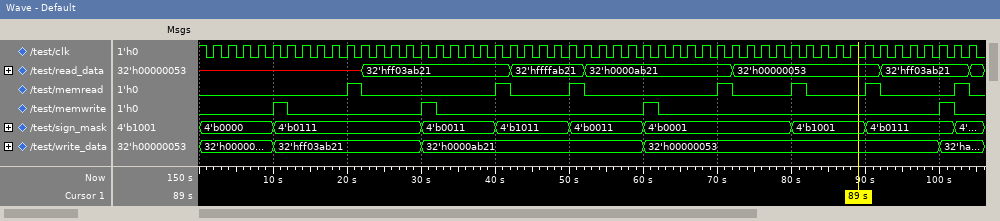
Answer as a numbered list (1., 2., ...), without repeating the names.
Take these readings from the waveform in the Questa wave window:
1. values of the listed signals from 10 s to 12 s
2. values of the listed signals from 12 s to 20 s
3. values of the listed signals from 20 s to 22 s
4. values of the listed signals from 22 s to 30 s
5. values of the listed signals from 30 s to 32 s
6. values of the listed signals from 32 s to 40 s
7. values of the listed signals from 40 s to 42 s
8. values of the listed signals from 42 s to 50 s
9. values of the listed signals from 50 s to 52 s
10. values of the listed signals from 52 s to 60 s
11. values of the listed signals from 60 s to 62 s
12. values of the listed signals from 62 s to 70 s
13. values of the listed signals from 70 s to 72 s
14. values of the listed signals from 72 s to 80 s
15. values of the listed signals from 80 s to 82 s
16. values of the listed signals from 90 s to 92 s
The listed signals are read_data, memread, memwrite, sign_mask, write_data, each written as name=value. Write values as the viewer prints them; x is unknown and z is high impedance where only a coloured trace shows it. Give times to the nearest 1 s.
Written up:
1. read_data=x, memread=0, memwrite=1, sign_mask=4'b0111, write_data=32'hff03ab21
2. read_data=x, memread=0, memwrite=0, sign_mask=4'b0111, write_data=32'hff03ab21
3. read_data=x, memread=1, memwrite=0, sign_mask=4'b0111, write_data=32'hff03ab21
4. read_data=32'hff03ab21, memread=0, memwrite=0, sign_mask=4'b0111, write_data=32'hff03ab21
5. read_data=32'hff03ab21, memread=0, memwrite=1, sign_mask=4'b0011, write_data=32'h0000ab21
6. read_data=32'hff03ab21, memread=0, memwrite=0, sign_mask=4'b0011, write_data=32'h0000ab21
7. read_data=32'hff03ab21, memread=1, memwrite=0, sign_mask=4'b1011, write_data=32'h0000ab21
8. read_data=32'hffffab21, memread=0, memwrite=0, sign_mask=4'b1011, write_data=32'h0000ab21
9. read_data=32'hffffab21, memread=1, memwrite=0, sign_mask=4'b0011, write_data=32'h0000ab21
10. read_data=32'h0000ab21, memread=0, memwrite=0, sign_mask=4'b0011, write_data=32'h0000ab21
11. read_data=32'h0000ab21, memread=0, memwrite=1, sign_mask=4'b0001, write_data=32'h00000053
12. read_data=32'h0000ab21, memread=0, memwrite=0, sign_mask=4'b0001, write_data=32'h00000053
13. read_data=32'h0000ab21, memread=1, memwrite=0, sign_mask=4'b0001, write_data=32'h00000053
14. read_data=32'h00000053, memread=0, memwrite=0, sign_mask=4'b0001, write_data=32'h00000053
15. read_data=32'h00000053, memread=1, memwrite=0, sign_mask=4'b1001, write_data=32'h00000053
16. read_data=32'h00000053, memread=1, memwrite=0, sign_mask=4'b0111, write_data=32'h00000053
